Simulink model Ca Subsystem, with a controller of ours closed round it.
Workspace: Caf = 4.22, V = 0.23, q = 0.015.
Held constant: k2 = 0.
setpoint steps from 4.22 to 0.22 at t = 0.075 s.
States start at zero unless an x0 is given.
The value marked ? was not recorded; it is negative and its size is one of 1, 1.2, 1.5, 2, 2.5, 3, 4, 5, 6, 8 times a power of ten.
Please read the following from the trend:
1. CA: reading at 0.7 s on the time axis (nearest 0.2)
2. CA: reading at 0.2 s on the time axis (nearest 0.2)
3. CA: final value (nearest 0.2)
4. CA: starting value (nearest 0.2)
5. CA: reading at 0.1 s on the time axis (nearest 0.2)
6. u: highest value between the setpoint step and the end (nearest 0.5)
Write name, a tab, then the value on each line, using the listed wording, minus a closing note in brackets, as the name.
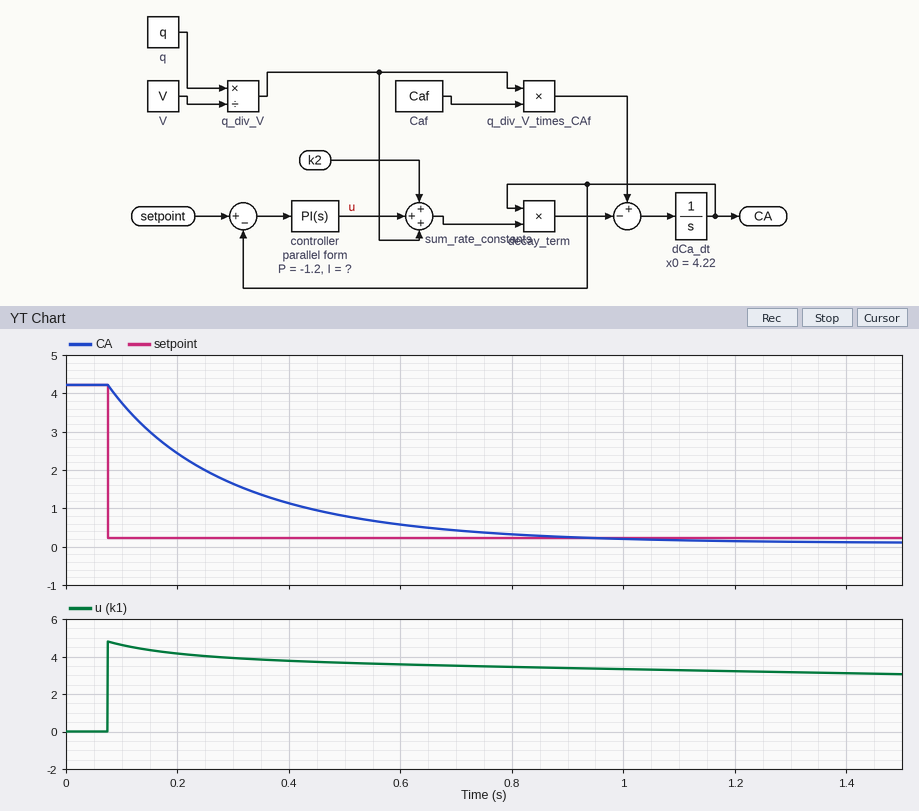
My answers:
CA: reading at 0.7 s on the time axis	0.4
CA: reading at 0.2 s on the time axis	2.4
CA: final value	0.2
CA: starting value	4.2
CA: reading at 0.1 s on the time axis	3.8
u: highest value between the setpoint step and the end	5.0
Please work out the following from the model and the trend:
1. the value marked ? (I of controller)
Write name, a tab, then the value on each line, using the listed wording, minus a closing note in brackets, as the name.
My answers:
the value marked ?	-4
